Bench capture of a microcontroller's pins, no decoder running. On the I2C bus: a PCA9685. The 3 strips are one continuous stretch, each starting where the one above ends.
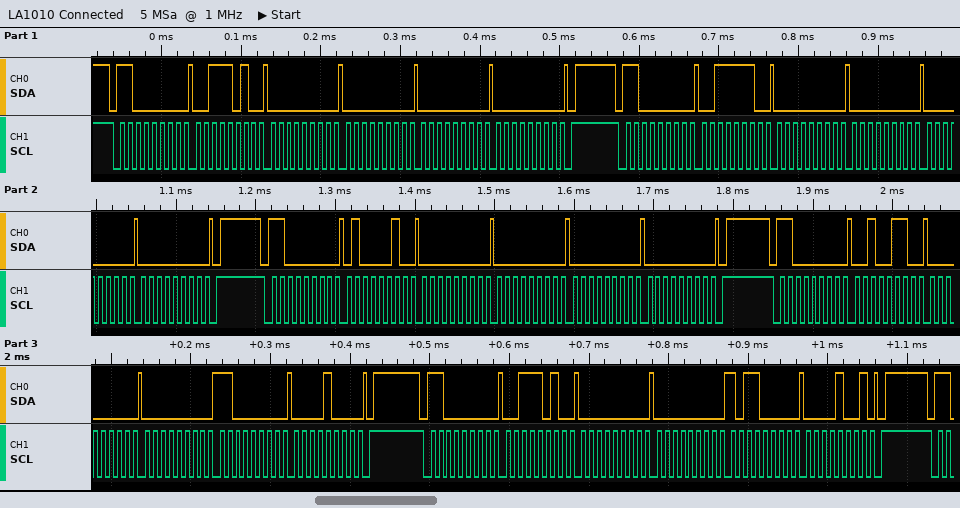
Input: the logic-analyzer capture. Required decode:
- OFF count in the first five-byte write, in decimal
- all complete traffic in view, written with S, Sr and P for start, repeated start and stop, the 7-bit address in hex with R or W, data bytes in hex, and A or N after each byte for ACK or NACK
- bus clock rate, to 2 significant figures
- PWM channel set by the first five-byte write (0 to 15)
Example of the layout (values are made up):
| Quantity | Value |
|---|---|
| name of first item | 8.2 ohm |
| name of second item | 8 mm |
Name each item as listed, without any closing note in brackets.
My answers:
| Quantity | Value |
|---|---|
| OFF count in the first five-byte write, in decimal | 0 |
| all complete traffic in view, written with S, Sr and P for start, repeated start and stop, the 7-bit address in hex with R or W, data bytes in hex, and A or N after each byte for ACK or NACK | S 60W A 3A A 00 A 00 A 00 A 00 A P S 60W A 3E A 00 A 00 A 00 A 00 A P S 60W A 42 A 00 A 00 A 00 A 00 A P S 60W A 26 A 00 A 00 A C0 A 08 A P S 60W A 3A A 00 A 00 A B0 A 09 A P |
| bus clock rate, to 2 significant figures | 100 kHz |
| PWM channel set by the first five-byte write | 13 |
